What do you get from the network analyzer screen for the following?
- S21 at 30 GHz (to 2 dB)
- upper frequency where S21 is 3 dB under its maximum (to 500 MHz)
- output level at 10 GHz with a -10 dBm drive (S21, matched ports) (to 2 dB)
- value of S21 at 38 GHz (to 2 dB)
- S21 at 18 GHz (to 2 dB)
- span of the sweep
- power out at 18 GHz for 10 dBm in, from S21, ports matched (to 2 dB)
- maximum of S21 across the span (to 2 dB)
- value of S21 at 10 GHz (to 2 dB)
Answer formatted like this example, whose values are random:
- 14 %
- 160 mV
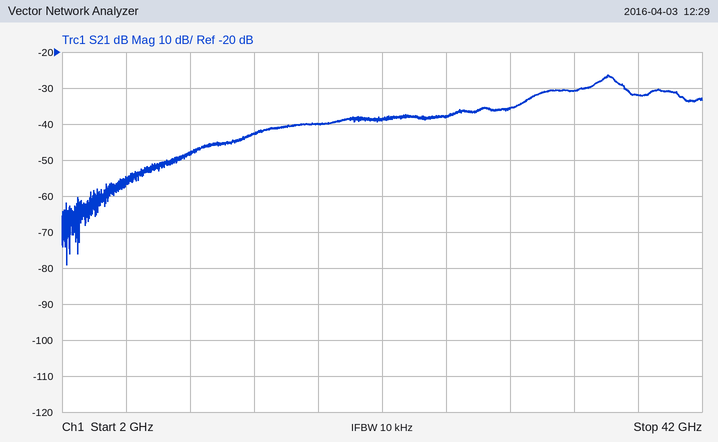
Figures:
- -36 dB
- 37.0 GHz
- -58 dBm
- -32 dB
- -40 dB
- 40 GHz
- -30 dBm
- -26 dB
- -48 dB
